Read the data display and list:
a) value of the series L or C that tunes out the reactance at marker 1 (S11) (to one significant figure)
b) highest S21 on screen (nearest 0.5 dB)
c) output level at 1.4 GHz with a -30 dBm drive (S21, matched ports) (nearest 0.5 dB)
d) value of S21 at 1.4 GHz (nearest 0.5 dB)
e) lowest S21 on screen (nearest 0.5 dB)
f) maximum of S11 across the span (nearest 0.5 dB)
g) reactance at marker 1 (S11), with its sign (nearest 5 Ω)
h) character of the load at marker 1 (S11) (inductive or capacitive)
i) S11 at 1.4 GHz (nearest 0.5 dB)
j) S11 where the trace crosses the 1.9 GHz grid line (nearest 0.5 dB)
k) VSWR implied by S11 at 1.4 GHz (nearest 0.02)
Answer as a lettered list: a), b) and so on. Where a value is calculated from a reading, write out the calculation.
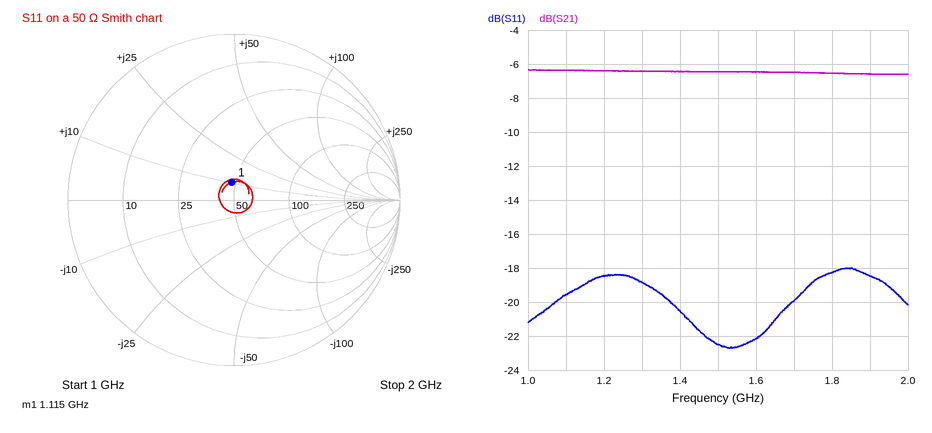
a) C = 1/(2π × 1.115 GHz × 10 Ω) ≈ 14.3 pF, so 10 pF to one significant figure
b) -6.5 dB
c) -30 dBm + (-6.5 dB) = -36.5 dBm
d) -6.5 dB
e) -6.5 dB
f) -18.0 dB
g) +10 Ω
h) inductive
i) -20.5 dB
j) -18.5 dB
k) |Γ| = 10^(-20.5/20) = 0.0944; VSWR = (1 + 0.0944)/(1 − 0.0944) ≈ 1.21, so 1.20 to the nearest 0.02
